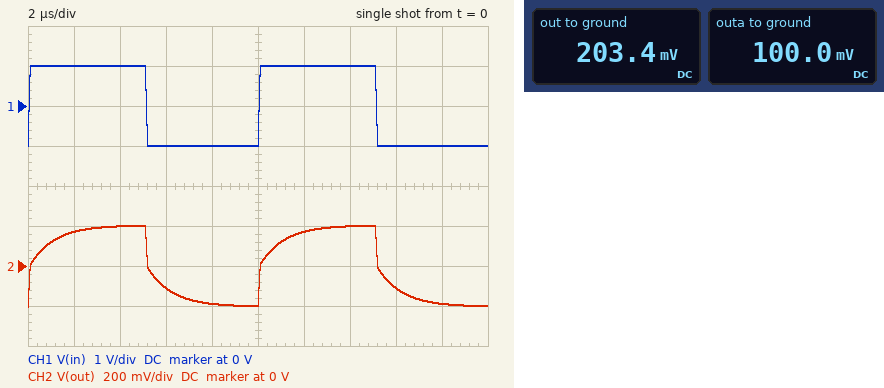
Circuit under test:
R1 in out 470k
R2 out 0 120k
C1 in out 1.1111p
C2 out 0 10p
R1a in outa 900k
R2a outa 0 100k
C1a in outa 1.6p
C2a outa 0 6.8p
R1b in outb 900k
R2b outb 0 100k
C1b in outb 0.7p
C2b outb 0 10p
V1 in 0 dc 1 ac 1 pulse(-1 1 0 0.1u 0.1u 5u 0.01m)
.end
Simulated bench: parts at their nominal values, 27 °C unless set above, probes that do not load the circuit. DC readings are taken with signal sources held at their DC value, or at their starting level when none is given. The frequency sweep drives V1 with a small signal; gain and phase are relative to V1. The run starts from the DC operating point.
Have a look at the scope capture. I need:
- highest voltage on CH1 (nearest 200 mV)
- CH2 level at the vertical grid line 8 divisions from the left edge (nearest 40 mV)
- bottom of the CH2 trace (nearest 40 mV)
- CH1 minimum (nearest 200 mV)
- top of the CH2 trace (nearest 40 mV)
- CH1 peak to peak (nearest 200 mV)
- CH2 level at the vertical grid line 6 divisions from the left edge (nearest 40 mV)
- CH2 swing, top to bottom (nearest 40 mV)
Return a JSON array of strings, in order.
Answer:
["1.0 V", "-120 mV", "-200 mV", "-1.0 V", "200 mV", "2.0 V", "160 mV", "400 mV"]
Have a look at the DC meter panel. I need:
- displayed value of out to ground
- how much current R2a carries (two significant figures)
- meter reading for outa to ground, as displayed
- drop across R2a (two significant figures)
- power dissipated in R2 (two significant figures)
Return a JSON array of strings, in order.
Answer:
["203.4 mV", "1.0 µA", "100.0 mV", "100 mV", "340 nW"]
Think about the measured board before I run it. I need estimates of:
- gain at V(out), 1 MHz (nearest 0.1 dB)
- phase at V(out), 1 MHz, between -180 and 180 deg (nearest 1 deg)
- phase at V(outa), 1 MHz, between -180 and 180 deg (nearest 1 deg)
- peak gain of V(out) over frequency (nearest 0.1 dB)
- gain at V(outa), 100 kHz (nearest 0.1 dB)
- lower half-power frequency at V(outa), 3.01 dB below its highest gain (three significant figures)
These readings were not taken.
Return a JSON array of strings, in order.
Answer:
["-19.7 dB", "-8 deg", "6 deg", "-13.8 dB", "-18.3 dB", "141 kHz"]
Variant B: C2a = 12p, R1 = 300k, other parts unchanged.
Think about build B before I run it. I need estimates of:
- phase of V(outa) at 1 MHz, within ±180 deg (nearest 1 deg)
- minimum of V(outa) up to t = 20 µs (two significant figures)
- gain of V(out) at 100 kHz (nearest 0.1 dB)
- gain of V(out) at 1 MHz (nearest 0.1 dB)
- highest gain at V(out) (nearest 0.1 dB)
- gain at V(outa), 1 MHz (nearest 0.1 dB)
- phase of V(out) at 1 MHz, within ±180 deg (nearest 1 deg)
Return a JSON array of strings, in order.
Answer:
["1 deg", "-130 mV", "-12.0 dB", "-19.2 dB", "-10.9 dB", "-18.6 dB", "-16 deg"]
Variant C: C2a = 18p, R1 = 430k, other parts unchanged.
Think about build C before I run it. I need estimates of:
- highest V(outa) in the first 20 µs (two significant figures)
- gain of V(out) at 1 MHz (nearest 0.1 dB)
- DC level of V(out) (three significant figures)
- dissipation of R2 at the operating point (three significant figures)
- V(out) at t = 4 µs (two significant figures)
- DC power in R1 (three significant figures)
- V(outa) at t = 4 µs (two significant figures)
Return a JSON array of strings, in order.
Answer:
["98 mV", "-19.6 dB", "218 mV", "397 nW", "210 mV", "1.42 µW", "96 mV"]
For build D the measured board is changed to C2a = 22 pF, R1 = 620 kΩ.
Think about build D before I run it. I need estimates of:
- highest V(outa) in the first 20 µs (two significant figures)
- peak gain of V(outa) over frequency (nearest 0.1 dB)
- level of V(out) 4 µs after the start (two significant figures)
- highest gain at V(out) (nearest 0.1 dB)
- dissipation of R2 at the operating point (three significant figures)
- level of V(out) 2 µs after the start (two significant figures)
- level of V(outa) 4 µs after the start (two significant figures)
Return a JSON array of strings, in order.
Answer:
["95 mV", "-20.0 dB", "160 mV", "-15.8 dB", "219 nW", "140 mV", "90 mV"]
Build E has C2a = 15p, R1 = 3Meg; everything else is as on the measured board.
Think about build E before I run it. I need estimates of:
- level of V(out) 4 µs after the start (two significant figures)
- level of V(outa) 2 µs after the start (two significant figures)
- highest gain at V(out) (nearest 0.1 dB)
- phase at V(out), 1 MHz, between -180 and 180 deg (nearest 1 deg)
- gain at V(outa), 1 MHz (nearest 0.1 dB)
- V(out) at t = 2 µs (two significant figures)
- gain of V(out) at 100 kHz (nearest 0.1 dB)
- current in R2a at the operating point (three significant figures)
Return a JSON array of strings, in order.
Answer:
["44 mV", "98 mV", "-20.0 dB", "4 deg", "-20.3 dB", "65 mV", "-23.2 dB", "1.00 µA"]
